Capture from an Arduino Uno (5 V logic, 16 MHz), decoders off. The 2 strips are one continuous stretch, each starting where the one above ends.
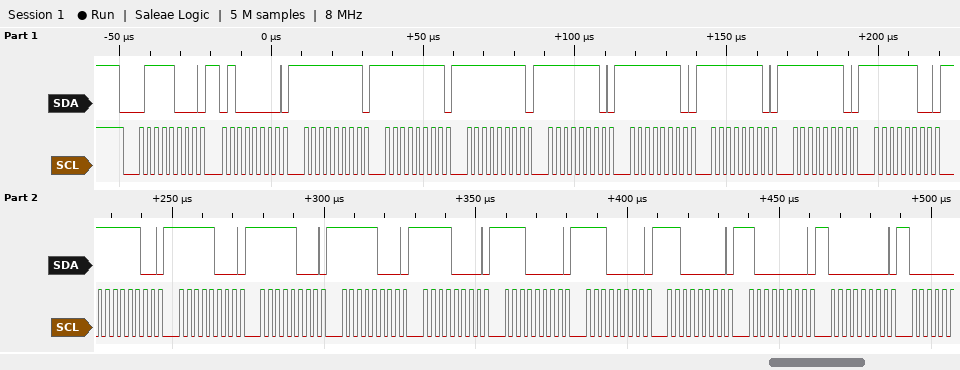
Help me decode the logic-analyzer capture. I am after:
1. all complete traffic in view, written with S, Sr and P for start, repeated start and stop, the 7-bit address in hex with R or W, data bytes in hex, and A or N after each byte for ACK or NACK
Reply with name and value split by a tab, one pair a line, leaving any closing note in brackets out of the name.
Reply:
all complete traffic in view, written with S, Sr and P for start, repeated start and stop, the 7-bit address in hex with R or W, data bytes in hex, and A or N after each byte for ACK or NACK	S 3CW A 40 A FF A FF A FF A FE A FE A FE A FE A FC A FC A F8 A F8 A F8 A F0 A E0 A E0 A C0 A 80 A 00 A
